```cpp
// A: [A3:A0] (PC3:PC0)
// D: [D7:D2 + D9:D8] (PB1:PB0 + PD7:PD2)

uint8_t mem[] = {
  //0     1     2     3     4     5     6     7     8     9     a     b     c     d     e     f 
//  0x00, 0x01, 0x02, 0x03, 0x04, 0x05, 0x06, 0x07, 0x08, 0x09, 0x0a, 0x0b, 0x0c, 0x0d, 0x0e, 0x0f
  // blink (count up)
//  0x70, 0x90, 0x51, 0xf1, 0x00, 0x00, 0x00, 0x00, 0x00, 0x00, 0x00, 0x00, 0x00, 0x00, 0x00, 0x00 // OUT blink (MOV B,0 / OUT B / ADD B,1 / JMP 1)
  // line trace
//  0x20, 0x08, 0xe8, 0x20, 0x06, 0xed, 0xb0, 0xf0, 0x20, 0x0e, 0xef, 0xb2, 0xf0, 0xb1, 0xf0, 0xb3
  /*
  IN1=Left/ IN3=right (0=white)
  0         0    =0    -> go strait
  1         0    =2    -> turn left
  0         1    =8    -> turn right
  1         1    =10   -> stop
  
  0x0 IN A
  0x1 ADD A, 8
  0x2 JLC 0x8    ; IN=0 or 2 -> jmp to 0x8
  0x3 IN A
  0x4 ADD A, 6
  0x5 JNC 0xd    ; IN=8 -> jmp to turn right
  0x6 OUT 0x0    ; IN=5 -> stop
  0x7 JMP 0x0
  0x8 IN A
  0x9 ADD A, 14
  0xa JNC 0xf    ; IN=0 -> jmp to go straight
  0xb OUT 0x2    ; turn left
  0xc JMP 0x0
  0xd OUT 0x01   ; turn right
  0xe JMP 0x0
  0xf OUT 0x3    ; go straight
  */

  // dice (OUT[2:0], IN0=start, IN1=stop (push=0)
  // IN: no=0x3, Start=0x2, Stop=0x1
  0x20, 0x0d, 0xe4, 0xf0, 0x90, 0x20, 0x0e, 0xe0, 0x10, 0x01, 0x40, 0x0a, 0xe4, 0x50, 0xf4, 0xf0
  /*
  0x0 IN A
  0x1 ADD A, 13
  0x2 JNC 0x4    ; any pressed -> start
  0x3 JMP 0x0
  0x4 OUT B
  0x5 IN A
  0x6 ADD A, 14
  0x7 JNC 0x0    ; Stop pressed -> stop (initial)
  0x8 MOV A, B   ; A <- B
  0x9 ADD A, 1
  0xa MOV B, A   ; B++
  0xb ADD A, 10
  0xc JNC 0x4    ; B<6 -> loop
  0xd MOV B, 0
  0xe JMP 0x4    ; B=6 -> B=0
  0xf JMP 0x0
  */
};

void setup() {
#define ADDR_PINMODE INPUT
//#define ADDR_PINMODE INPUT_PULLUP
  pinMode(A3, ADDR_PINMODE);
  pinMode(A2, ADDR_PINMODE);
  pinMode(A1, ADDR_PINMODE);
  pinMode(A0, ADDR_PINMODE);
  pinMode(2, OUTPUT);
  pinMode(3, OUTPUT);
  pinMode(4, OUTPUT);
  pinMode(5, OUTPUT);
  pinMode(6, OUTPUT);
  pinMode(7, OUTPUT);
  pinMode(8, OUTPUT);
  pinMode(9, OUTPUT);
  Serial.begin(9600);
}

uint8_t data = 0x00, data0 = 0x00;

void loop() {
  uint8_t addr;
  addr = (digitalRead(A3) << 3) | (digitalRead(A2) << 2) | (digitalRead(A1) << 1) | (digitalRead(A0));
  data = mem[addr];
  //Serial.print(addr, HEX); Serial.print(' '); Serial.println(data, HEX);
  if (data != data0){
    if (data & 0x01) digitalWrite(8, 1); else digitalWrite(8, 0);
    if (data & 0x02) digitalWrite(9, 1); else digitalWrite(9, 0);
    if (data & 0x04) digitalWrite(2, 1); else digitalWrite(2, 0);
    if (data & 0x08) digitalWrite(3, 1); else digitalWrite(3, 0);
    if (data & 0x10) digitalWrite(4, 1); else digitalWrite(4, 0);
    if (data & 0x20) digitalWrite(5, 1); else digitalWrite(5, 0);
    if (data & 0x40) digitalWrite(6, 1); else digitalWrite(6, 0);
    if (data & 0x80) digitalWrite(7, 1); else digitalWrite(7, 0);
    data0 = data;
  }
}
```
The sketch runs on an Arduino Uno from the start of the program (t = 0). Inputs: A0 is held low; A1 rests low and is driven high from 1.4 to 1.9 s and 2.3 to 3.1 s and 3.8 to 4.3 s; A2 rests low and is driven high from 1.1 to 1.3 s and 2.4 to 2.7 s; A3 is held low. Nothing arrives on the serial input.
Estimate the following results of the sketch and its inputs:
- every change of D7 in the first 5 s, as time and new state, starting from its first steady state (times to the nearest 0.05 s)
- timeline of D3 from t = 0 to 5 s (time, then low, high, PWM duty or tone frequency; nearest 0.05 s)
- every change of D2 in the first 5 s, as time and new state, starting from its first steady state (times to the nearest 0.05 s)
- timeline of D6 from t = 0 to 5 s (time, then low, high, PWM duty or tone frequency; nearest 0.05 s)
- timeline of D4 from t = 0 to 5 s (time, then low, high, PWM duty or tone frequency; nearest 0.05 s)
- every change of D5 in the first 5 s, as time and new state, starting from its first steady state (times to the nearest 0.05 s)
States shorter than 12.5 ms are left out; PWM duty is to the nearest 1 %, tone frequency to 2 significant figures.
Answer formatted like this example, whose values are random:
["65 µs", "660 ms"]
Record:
["0 s low; 1.1 s high; 1.3 s low; 1.4 s high; 1.9 s low; 2.3 s high; 2.4 s low; 2.7 s high; 3.1 s low; 3.8 s high; 4.3 s low", "0 s low; 2.4 s high; 2.7 s low", "0 s low; 1.4 s high; 1.9 s low; 2.3 s high; 3.1 s low; 3.8 s high; 4.3 s low", "0 s low; 1.4 s high; 1.9 s low; 2.3 s high; 2.4 s low; 2.7 s high; 3.1 s low; 3.8 s high; 4.3 s low", "0 s low; 1.1 s high; 1.3 s low", "0 s high; 1.1 s low; 1.3 s high; 2.4 s low; 2.7 s high"]
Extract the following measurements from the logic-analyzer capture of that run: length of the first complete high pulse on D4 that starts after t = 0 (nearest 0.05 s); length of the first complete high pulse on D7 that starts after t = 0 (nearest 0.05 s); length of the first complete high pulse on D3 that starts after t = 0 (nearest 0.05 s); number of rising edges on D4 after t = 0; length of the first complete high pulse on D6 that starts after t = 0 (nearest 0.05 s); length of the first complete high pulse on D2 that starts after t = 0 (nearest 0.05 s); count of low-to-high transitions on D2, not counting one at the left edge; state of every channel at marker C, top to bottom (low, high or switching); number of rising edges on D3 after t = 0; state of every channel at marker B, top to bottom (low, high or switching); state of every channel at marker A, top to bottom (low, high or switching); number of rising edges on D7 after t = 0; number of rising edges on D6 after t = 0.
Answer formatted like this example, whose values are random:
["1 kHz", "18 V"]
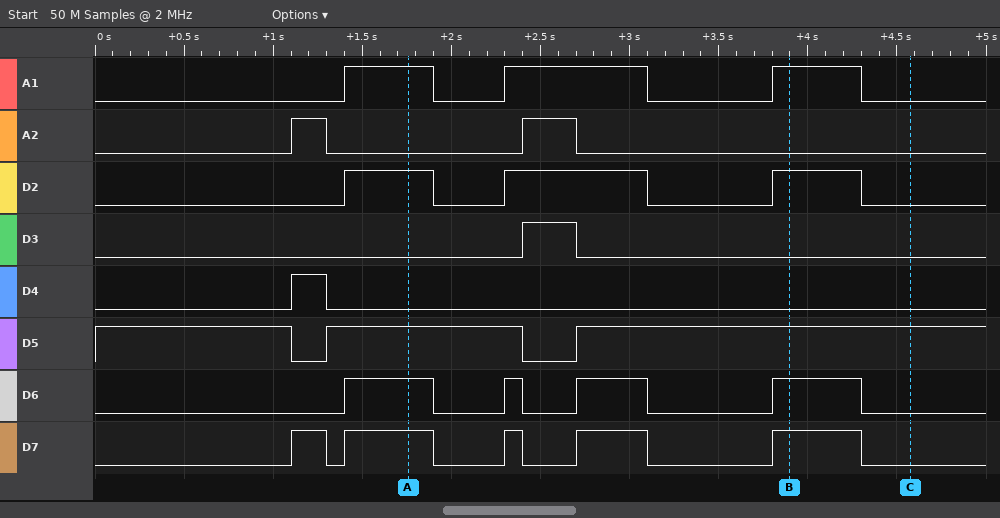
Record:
["0.20 s", "0.20 s", "0.30 s", "1", "0.50 s", "0.50 s", "3", "A1 low, A2 low, D2 low, D3 low, D4 low, D5 high, D6 low, D7 low", "1", "A1 high, A2 low, D2 high, D3 low, D4 low, D5 high, D6 high, D7 high", "A1 high, A2 low, D2 high, D3 low, D4 low, D5 high, D6 high, D7 high", "5", "4"]
